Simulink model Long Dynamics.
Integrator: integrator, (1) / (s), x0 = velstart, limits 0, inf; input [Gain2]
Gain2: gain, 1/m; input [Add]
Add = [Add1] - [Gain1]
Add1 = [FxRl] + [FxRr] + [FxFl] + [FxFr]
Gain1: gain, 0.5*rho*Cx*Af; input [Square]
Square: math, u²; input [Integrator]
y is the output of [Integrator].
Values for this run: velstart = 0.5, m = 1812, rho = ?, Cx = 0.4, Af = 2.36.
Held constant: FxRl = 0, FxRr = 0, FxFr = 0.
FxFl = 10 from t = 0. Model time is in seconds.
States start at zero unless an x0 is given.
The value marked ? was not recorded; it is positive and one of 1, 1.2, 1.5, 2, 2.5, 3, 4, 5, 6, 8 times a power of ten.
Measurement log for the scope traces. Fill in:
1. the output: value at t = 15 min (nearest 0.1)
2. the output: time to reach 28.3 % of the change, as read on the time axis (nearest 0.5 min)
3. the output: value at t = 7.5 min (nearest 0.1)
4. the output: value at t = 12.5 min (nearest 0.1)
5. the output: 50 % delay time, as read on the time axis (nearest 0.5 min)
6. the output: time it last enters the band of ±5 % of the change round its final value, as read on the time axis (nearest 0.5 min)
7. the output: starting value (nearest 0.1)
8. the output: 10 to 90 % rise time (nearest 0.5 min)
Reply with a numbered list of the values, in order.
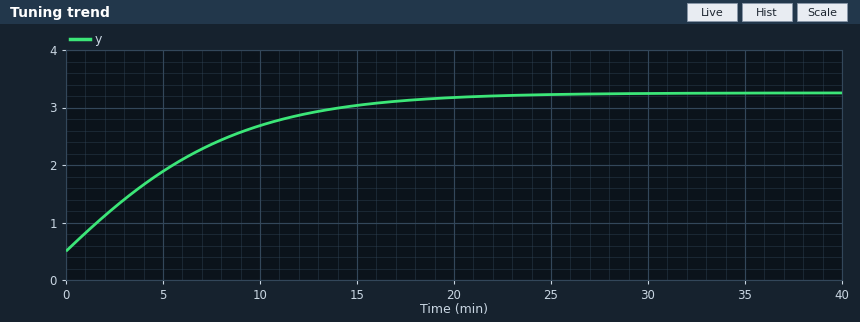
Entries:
1. 3.0
2. 2.5 min
3. 2.4
4. 2.9
5. 5.0 min
6. 17.5 min
7. 0.5
8. 13.0 min
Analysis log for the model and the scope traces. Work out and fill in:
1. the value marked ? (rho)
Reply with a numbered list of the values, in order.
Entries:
1. 2
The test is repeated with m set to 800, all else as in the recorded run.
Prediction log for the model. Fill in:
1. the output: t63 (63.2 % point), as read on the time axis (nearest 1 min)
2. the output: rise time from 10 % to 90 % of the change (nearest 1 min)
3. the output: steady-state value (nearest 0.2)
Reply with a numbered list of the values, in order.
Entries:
1. 3 min
2. 6 min
3. 3.2
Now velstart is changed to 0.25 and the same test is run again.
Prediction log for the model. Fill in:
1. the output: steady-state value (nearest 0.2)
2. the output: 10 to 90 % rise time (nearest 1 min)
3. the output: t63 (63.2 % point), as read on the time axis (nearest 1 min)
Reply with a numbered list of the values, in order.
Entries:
1. 3.2
2. 13 min
3. 7 min
